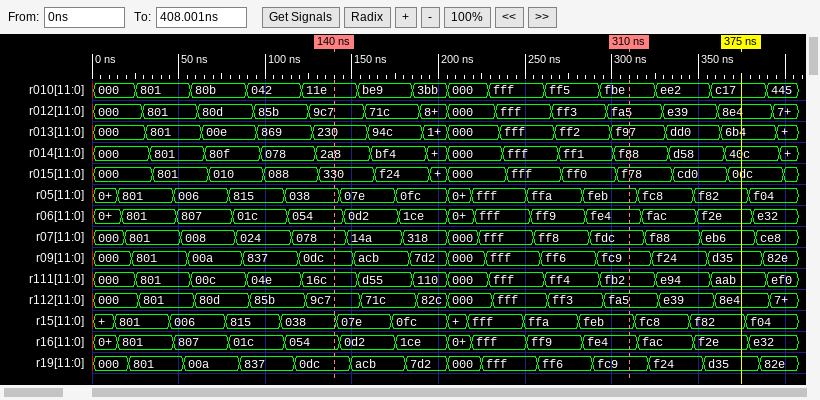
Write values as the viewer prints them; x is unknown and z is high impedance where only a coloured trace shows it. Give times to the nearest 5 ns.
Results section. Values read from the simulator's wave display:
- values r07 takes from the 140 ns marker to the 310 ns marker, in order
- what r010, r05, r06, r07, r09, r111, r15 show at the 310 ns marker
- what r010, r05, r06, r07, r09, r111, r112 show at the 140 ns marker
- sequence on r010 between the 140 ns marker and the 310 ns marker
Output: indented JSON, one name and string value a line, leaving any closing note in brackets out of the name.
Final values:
{
  "values r07 takes from the 140 ns marker to the 310 ns marker, in order": "078, 14a, 318, 000, fff, ff8, fdc",
  "what r010, r05, r06, r07, r09, r111, r15 show at the 310 ns marker": "r010=fbe, r05=feb, r06=fe4, r07=fdc, r09=fc9, r111=fb2, r15=feb",
  "what r010, r05, r06, r07, r09, r111, r112 show at the 140 ns marker": "r010=11e, r05=038, r06=054, r07=078, r09=0dc, r111=16c, r112=9c7",
  "sequence on r010 between the 140 ns marker and the 310 ns marker": "11e, be9, 3bb, 000, fff, ff5, fbe"
}
